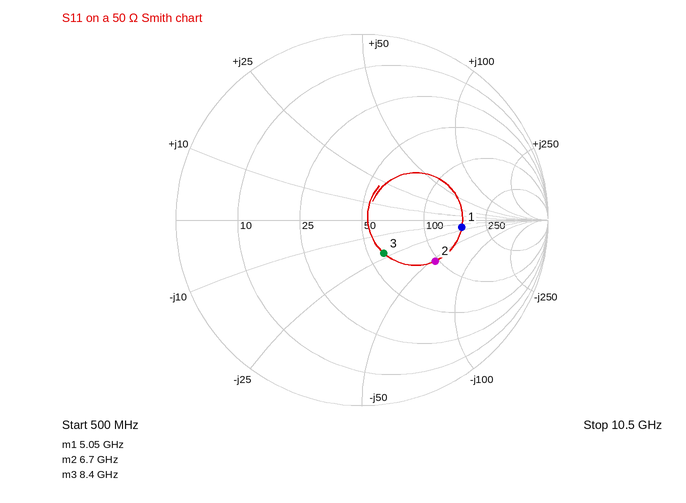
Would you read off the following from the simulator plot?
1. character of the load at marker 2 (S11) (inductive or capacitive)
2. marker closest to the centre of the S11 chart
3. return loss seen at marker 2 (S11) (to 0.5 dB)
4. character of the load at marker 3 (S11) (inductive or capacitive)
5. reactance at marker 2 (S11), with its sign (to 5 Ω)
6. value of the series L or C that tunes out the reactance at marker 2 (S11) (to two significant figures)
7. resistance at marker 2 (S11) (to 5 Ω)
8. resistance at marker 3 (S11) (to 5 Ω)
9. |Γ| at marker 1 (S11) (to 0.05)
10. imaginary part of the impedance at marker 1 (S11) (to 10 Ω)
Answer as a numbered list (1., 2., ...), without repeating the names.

1. capacitive
2. marker 3
3. 7.0 dB
4. capacitive
5. -55 Ω
6. 1.3 nH
7. 95 Ω
8. 60 Ω
9. 0.55
10. -20 Ω
